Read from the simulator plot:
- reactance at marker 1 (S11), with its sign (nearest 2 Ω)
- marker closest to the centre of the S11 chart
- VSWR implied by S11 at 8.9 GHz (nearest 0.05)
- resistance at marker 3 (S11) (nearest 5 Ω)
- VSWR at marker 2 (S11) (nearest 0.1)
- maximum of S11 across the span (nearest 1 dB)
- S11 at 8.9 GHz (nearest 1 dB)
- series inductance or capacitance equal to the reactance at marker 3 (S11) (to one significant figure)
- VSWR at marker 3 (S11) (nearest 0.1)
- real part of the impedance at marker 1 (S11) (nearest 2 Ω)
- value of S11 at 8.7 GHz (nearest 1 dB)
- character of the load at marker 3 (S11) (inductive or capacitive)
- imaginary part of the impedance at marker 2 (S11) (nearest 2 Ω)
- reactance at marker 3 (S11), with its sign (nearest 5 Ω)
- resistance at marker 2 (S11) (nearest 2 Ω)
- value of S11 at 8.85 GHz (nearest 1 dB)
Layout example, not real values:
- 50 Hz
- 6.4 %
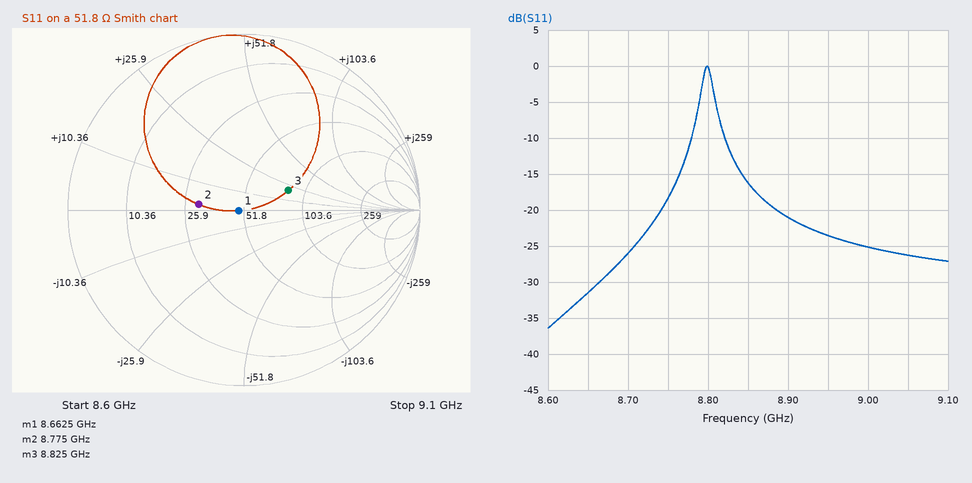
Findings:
- 0 Ω
- marker 1
- 1.20
- 85 Ω
- 1.7
- 0 dB
- -21 dB
- 400 pH
- 1.8
- 48 Ω
- -26 dB
- inductive
- +2 Ω
- +20 Ω
- 30 Ω
- -16 dB
